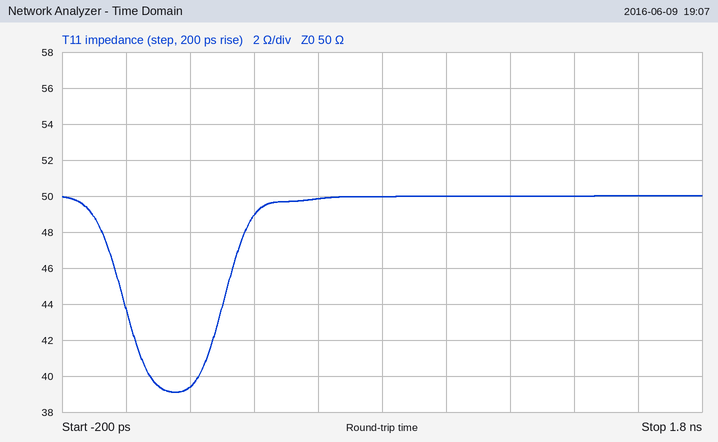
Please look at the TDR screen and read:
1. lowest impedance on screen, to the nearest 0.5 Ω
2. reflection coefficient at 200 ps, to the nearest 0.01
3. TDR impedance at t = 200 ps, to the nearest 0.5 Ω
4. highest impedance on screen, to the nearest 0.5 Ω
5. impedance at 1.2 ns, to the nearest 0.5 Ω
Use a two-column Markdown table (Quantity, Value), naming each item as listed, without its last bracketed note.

| Quantity | Value |
|---|---|
| lowest impedance on screen, to the nearest 0.5 Ω | 39.0 Ω |
| reflection coefficient at 200 ps, to the nearest 0.01 | -0.12 |
| TDR impedance at t = 200 ps, to the nearest 0.5 Ω | 39.5 Ω |
| highest impedance on screen, to the nearest 0.5 Ω | 50.0 Ω |
| impedance at 1.2 ns, to the nearest 0.5 Ω | 50.0 Ω |
